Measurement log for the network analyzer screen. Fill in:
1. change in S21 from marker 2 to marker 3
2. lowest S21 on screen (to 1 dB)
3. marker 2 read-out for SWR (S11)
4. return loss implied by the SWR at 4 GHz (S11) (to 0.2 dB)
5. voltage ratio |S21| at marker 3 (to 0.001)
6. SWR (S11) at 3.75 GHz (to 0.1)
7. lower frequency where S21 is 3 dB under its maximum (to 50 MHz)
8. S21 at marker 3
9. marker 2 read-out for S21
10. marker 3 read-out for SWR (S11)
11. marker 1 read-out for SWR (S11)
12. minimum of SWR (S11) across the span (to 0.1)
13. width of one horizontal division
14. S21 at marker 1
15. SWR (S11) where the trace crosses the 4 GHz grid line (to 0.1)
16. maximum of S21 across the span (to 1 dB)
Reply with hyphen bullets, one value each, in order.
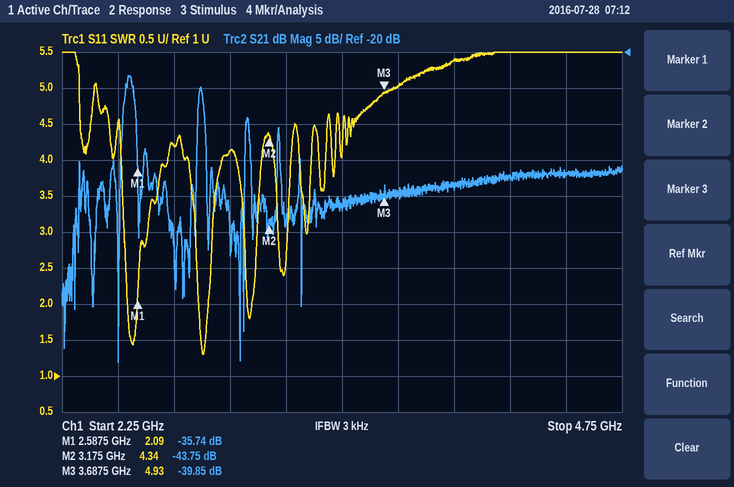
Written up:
- 3.90 dB
- -63 dB
- 4.34
- 3.2 dB
- 0.010
- 5.0
- 2.55 GHz
- -39.85 dB
- -43.75 dB
- 4.93
- 2.09
- 1.3
- 250 MHz
- -35.74 dB
- 5.4
- -23 dB
